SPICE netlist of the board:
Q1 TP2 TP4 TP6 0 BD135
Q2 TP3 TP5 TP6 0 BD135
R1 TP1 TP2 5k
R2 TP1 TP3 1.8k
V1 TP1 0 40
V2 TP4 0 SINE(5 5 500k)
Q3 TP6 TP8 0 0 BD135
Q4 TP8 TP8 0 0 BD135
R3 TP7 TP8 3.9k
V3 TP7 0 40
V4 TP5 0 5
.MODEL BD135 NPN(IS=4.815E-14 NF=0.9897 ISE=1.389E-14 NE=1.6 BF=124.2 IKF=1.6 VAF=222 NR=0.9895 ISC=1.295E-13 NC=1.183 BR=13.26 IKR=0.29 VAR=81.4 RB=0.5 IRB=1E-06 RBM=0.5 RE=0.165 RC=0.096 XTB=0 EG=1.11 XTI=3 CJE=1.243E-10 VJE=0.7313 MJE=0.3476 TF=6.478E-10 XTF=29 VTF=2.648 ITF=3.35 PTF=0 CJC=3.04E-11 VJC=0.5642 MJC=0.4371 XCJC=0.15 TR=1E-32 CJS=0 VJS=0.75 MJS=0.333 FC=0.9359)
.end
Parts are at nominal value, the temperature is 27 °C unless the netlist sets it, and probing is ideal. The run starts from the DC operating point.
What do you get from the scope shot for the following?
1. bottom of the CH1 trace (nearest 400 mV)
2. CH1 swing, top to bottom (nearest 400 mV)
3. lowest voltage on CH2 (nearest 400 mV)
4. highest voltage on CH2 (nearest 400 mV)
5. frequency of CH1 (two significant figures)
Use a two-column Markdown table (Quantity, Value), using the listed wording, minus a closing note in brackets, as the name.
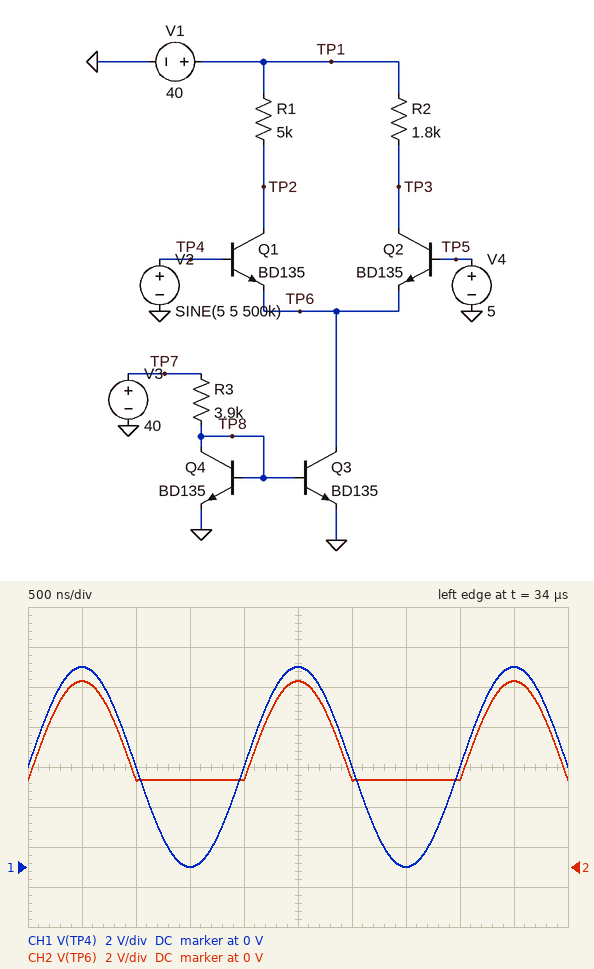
| Quantity | Value |
|---|---|
| bottom of the CH1 trace | 0 V |
| CH1 swing, top to bottom | 10.0 V |
| lowest voltage on CH2 | 4.4 V |
| highest voltage on CH2 | 9.2 V |
| frequency of CH1 | 500 kHz |
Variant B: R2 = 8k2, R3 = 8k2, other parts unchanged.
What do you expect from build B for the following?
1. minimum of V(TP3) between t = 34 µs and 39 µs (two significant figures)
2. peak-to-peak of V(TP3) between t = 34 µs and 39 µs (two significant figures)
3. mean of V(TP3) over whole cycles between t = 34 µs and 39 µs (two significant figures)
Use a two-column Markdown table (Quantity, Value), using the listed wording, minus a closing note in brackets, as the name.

| Quantity | Value |
|---|---|
| minimum of V(TP3) between t = 34 µs and 39 µs | 4.3 V |
| peak-to-peak of V(TP3) between t = 34 µs and 39 µs | 36 V |
| mean of V(TP3) over whole cycles between t = 34 µs and 39 µs | 22 V |
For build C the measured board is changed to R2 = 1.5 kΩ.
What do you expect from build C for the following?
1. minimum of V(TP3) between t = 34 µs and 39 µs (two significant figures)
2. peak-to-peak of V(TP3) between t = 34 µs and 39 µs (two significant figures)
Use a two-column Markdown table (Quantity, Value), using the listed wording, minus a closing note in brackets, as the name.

| Quantity | Value |
|---|---|
| minimum of V(TP3) between t = 34 µs and 39 µs | 22 V |
| peak-to-peak of V(TP3) between t = 34 µs and 39 µs | 18 V |
